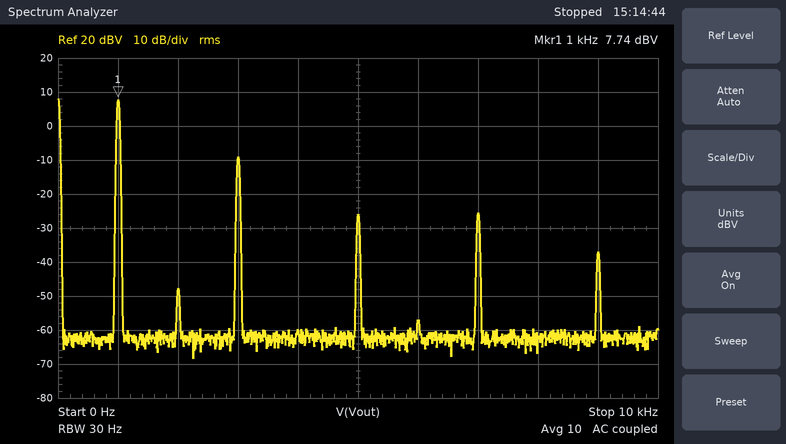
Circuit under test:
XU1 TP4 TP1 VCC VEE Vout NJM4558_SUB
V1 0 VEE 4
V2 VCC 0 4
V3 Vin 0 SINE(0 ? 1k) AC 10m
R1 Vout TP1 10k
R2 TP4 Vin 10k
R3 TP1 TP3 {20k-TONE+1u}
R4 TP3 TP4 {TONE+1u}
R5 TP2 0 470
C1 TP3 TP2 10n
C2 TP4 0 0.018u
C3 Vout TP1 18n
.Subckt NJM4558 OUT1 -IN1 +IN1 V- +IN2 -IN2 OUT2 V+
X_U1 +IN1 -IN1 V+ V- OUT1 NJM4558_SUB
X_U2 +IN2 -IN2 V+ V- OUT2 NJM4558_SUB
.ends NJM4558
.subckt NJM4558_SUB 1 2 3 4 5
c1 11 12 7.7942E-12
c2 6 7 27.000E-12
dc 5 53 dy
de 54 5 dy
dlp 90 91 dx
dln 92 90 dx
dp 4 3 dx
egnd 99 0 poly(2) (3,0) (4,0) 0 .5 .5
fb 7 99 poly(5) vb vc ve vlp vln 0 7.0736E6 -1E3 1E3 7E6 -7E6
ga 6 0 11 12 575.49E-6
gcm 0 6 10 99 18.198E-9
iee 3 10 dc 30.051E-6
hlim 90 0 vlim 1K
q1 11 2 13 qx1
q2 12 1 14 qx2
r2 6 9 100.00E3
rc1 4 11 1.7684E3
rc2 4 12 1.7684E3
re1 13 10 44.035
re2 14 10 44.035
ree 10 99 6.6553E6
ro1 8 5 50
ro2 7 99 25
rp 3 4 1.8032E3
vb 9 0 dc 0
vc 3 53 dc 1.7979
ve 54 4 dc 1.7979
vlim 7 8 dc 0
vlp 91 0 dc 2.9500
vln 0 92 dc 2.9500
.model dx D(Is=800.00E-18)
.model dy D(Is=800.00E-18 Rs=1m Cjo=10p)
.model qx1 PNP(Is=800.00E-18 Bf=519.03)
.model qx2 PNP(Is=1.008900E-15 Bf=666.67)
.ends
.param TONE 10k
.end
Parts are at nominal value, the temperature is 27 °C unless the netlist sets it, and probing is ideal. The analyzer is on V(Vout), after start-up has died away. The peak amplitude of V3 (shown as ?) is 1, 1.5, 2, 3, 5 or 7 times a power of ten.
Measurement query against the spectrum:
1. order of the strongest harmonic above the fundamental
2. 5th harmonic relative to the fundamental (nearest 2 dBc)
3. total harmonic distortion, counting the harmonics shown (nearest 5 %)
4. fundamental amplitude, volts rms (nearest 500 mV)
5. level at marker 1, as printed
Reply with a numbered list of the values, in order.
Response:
1. 3
2. -34 dBc
3. 15 %
4. 2.5 V
5. 7.74 dBV
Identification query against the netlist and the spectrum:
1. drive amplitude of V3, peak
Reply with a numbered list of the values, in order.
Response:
1. 7 V
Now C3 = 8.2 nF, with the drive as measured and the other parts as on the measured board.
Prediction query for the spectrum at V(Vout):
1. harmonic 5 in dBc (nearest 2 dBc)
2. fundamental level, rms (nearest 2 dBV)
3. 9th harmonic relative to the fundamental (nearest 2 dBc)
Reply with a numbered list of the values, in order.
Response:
1. -36 dBc
2. 8 dBV
3. -48 dBc
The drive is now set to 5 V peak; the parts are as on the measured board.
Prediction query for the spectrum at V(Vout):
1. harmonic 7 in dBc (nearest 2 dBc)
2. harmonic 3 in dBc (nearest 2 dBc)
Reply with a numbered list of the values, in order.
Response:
1. -38 dBc
2. -30 dBc
